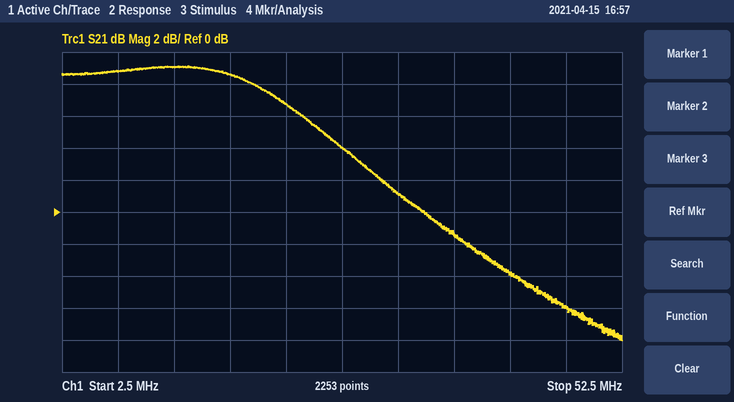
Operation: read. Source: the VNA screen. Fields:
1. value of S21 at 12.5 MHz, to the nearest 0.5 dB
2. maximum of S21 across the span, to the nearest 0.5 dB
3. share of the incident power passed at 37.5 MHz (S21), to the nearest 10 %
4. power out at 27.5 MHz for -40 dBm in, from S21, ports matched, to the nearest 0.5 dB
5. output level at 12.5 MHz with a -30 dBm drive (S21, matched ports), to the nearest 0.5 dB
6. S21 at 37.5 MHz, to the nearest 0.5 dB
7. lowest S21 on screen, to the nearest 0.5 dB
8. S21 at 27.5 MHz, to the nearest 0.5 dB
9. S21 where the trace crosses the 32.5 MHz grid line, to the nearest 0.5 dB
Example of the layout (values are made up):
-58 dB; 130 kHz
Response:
9.0 dB; 9.0 dB; 70 %; -36.0 dBm; -21.0 dBm; -1.5 dB; -8.0 dB; 4.0 dB; 1.0 dB
